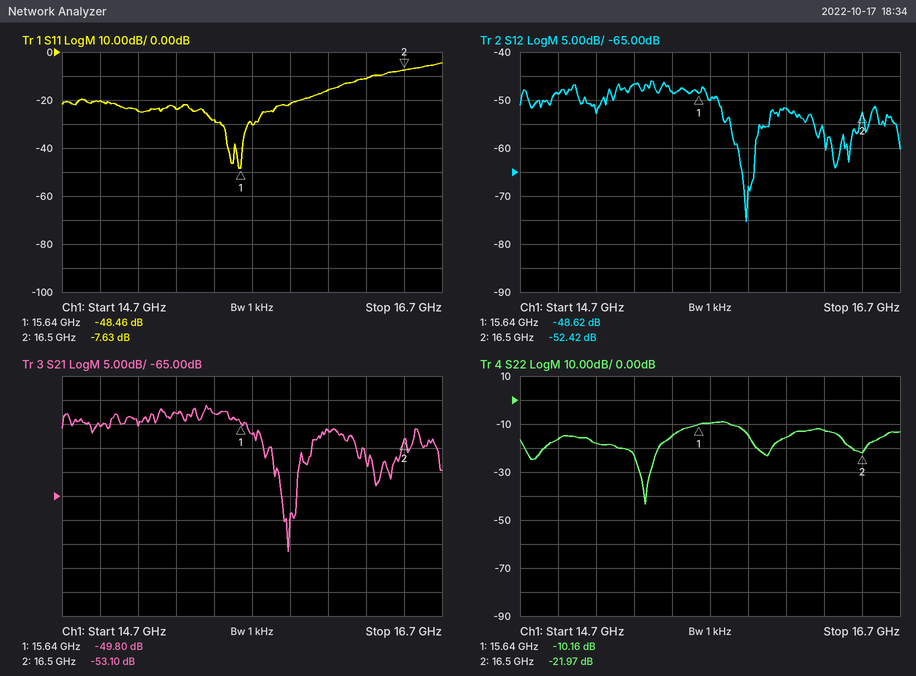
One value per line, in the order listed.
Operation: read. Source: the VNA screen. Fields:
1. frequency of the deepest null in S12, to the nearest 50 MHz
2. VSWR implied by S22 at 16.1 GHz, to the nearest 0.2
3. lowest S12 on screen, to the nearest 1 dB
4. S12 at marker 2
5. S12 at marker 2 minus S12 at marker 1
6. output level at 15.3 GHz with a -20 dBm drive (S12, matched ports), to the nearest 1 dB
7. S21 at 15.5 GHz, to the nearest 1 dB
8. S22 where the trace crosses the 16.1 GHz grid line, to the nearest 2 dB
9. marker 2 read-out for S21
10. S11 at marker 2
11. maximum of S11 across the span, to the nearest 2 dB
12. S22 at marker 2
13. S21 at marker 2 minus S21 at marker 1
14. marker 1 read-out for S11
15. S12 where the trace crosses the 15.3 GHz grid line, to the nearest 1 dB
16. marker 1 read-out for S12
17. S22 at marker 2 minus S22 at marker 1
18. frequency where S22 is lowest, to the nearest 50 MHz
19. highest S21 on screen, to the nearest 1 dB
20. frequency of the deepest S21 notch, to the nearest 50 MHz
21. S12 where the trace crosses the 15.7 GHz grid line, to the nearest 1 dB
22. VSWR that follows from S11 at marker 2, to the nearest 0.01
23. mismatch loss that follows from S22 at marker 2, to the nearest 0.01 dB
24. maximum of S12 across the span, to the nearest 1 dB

15.90 GHz
1.4
-75 dB
-52.42 dB
-3.80 dB
-67 dBm
-48 dB
-16 dB
-53.10 dB
-7.63 dB
-4 dB
-21.97 dB
-3.30 dB
-48.46 dB
-47 dB
-48.62 dB
-11.81 dB
15.35 GHz
-46 dB
15.90 GHz
-50 dB
2.42
0.03 dB
-46 dB
